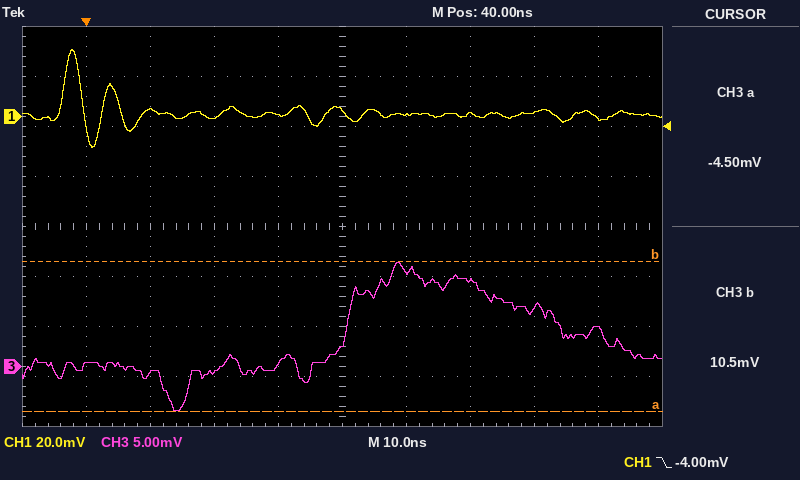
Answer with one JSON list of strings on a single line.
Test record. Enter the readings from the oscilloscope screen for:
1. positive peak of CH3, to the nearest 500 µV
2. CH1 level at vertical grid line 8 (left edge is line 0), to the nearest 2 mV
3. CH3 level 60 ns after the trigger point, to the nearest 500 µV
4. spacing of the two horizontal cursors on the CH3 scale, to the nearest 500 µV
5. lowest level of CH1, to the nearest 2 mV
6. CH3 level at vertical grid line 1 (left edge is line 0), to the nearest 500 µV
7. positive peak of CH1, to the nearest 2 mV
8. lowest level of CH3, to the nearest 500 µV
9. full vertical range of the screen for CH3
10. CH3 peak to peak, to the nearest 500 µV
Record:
["10.5 mV", "2 mV", "8.5 mV", "15.0 mV", "-12 mV", "0.0 mV", "26 mV", "-4.5 mV", "40 mV", "15.0 mV"]
